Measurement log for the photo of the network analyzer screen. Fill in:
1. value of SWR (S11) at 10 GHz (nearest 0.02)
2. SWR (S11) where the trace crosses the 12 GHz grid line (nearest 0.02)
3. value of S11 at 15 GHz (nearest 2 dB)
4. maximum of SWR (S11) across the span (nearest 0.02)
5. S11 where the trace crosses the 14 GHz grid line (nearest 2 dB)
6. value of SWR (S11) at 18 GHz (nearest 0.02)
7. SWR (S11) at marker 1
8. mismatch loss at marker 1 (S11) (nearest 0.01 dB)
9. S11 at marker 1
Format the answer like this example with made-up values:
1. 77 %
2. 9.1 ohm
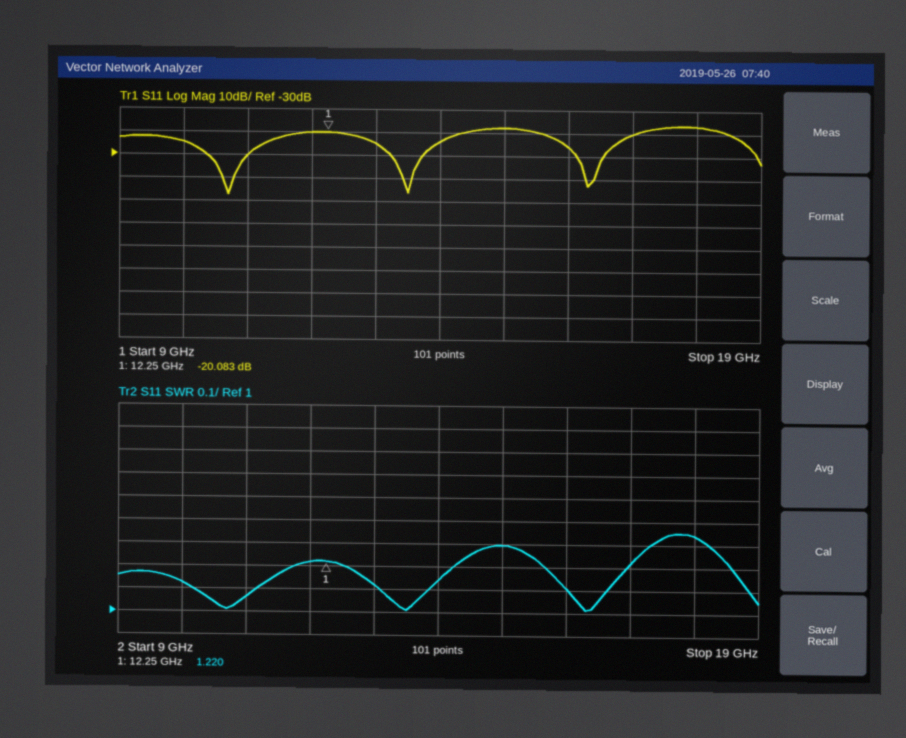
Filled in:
1. 1.12
2. 1.22
3. -18 dB
4. 1.36
5. -24 dB
6. 1.34
7. 1.220
8. 0.04 dB
9. -20.083 dB
